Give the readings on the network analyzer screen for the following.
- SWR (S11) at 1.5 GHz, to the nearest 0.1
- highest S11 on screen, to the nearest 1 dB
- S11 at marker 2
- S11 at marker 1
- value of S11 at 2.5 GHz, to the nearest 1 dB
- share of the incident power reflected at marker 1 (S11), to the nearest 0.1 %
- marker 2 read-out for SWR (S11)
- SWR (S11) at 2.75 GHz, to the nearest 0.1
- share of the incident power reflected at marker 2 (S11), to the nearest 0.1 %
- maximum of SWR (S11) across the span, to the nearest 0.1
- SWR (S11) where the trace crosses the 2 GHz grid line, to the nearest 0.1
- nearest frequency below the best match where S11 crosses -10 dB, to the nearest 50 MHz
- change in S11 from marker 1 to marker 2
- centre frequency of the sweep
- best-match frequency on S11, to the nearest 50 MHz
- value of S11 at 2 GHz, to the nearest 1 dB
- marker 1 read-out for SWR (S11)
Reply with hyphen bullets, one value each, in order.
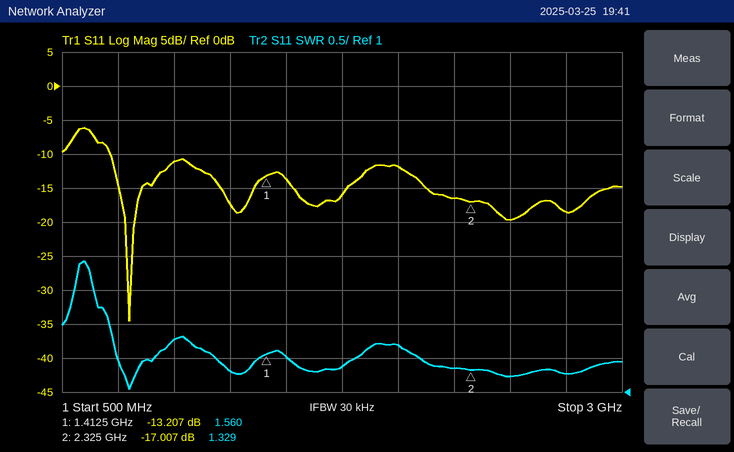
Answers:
- 1.5
- -6 dB
- -17.007 dB
- -13.207 dB
- -20 dB
- 4.8 %
- 1.329
- 1.3
- 2.0 %
- 2.9
- 1.7
- 700 MHz
- -3.800 dB
- 1.75 GHz
- 800 MHz
- -12 dB
- 1.560
